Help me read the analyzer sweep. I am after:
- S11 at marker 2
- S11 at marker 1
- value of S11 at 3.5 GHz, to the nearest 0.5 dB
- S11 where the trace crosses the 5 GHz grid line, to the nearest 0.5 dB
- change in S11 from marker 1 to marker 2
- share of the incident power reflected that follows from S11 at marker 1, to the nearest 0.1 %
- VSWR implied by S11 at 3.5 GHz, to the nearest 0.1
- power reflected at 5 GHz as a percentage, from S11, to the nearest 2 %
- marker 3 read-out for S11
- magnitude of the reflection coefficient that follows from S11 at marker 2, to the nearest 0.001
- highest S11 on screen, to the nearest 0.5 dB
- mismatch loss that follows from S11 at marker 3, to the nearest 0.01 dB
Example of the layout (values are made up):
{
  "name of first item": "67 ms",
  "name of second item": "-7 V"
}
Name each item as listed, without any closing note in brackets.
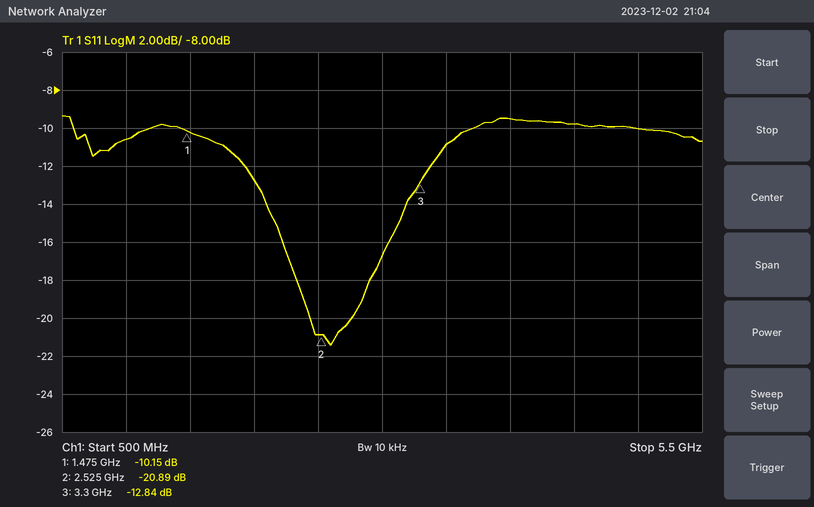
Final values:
{
  "S11 at marker 2": "-20.89 dB",
  "S11 at marker 1": "-10.15 dB",
  "value of S11 at 3.5 GHz, to the nearest 0.5 dB": "-11.0 dB",
  "S11 where the trace crosses the 5 GHz grid line, to the nearest 0.5 dB": "-10.0 dB",
  "change in S11 from marker 1 to marker 2": "-10.74 dB",
  "share of the incident power reflected that follows from S11 at marker 1, to the nearest 0.1 %": "9.7 %",
  "VSWR implied by S11 at 3.5 GHz, to the nearest 0.1": "1.8",
  "power reflected at 5 GHz as a percentage, from S11, to the nearest 2 %": "10 %",
  "marker 3 read-out for S11": "-12.84 dB",
  "magnitude of the reflection coefficient that follows from S11 at marker 2, to the nearest 0.001": "0.090",
  "highest S11 on screen, to the nearest 0.5 dB": "-9.5 dB",
  "mismatch loss that follows from S11 at marker 3, to the nearest 0.01 dB": "0.23 dB"
}
